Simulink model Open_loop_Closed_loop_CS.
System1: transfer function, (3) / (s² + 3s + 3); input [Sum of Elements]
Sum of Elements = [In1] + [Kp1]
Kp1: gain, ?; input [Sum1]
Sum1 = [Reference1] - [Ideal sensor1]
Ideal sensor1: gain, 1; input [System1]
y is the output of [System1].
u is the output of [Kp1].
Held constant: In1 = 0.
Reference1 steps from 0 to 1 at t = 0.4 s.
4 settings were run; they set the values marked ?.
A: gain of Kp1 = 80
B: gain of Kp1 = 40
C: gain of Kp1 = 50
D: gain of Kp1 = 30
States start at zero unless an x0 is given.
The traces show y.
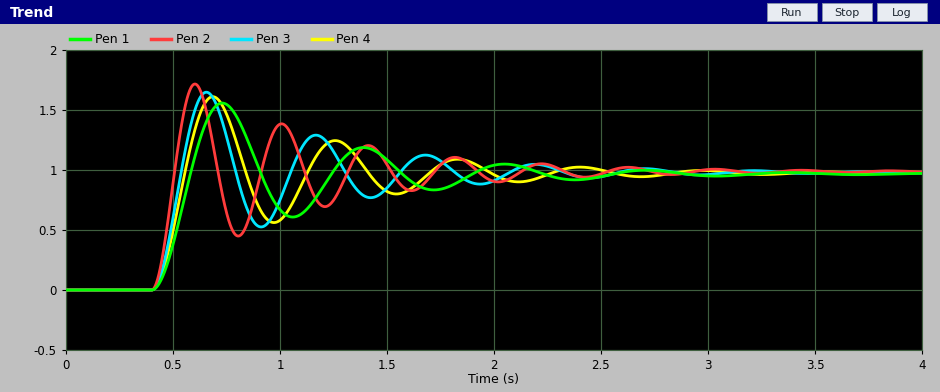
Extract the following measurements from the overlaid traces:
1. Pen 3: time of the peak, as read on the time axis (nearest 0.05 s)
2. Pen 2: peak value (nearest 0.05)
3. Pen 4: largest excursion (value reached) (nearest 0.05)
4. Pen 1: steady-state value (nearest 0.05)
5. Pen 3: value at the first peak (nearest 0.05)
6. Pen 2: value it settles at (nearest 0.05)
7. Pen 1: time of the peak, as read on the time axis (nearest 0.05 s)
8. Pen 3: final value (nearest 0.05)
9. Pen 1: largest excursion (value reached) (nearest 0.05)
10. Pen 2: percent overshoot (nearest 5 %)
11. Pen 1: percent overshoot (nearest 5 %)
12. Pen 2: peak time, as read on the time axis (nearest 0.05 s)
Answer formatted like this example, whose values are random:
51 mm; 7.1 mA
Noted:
0.65 s; 1.70; 1.60; 0.95; 1.65; 1.00; 0.75 s; 1.00; 1.55; 75 %; 60 %; 0.60 s
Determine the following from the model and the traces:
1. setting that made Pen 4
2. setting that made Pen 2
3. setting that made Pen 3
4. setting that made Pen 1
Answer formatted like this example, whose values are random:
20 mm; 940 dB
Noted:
B; A; C; D
